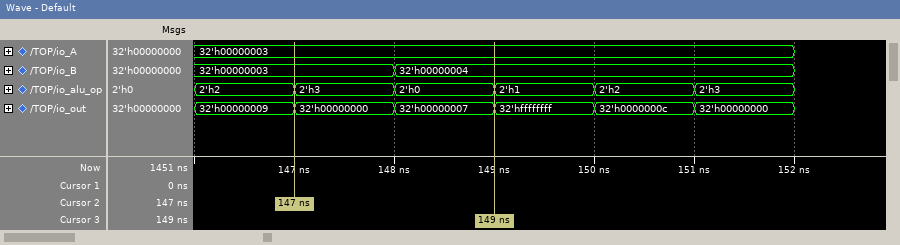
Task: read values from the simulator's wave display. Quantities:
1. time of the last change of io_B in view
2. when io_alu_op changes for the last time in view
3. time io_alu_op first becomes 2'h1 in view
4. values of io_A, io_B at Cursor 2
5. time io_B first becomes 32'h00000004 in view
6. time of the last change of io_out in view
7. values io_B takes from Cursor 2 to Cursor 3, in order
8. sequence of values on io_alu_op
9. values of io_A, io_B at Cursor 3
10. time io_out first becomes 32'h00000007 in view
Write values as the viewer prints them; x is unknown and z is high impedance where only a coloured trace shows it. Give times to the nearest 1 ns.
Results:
148 ns
151 ns
149 ns
io_A=32'h00000003, io_B=32'h00000003
148 ns
151 ns
32'h00000003, 32'h00000004
2'h2, 2'h3, 2'h0, 2'h1, 2'h2, 2'h3
io_A=32'h00000003, io_B=32'h00000004
148 ns
